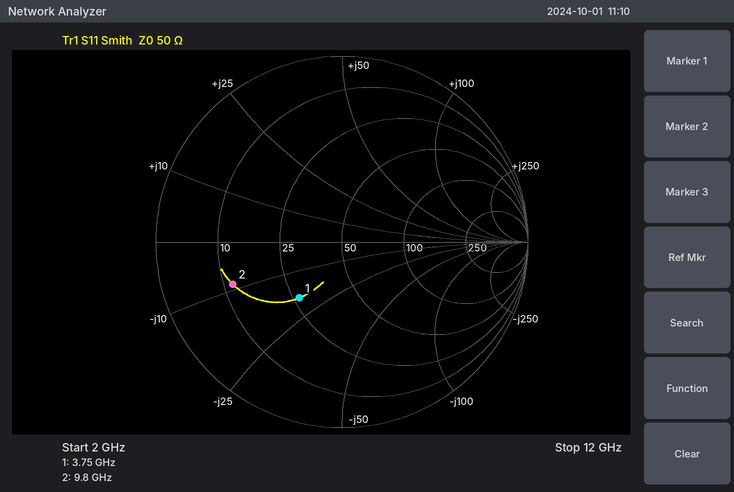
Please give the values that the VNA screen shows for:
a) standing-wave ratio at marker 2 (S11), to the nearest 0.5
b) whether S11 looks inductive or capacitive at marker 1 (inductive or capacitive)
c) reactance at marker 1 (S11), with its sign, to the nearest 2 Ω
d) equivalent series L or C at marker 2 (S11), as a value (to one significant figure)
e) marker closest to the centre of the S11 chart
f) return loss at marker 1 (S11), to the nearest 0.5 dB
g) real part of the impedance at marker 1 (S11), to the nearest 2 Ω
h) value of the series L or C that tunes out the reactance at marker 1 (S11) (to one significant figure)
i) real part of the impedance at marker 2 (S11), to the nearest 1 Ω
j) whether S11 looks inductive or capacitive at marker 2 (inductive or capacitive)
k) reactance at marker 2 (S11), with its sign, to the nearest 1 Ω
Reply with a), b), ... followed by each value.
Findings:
a) 4.5
b) capacitive
c) -18 Ω
d) 2 pF
e) marker 1
f) 8.5 dB
g) 26 Ω
h) 800 pH
i) 12 Ω
j) capacitive
k) -9 Ω
